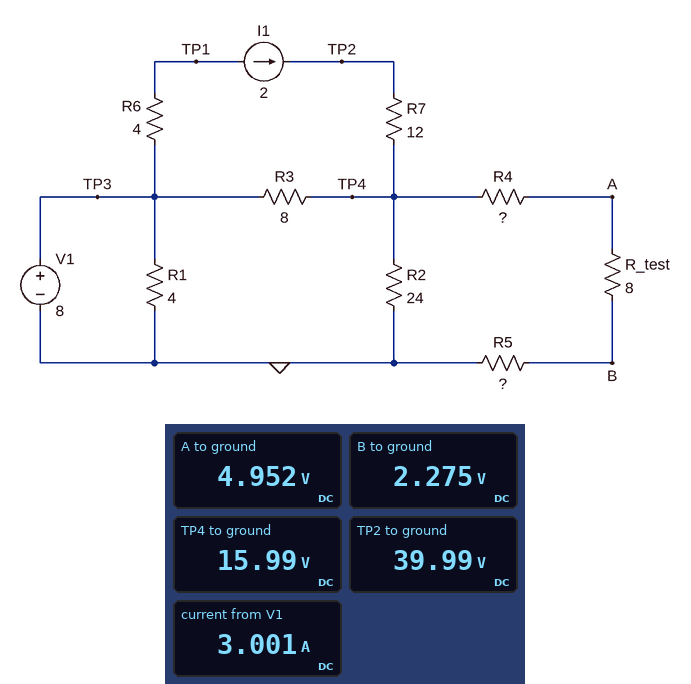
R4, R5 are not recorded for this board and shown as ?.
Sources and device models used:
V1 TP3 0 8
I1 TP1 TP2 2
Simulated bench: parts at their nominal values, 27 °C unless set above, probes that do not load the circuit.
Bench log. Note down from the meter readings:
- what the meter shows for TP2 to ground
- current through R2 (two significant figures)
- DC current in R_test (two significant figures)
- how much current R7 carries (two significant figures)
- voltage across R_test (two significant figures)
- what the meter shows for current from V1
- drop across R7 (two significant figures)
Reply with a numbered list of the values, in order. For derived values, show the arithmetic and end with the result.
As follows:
1. 39.99 V
2. (15.99 V) / 24 Ω = 670 mA
3. (4.952 V - 2.275 V) / 8 Ω = 330 mA
4. (39.99 V - 15.99 V) / 12 Ω = 2.0 A
5. 4.952 V - 2.275 V = 2.7 V
6. 3.001 A
7. 39.99 V - 15.99 V = 24 V
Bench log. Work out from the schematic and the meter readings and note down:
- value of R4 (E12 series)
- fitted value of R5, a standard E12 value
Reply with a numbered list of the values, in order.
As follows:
1. 33 Ω
2. 6.8 Ω
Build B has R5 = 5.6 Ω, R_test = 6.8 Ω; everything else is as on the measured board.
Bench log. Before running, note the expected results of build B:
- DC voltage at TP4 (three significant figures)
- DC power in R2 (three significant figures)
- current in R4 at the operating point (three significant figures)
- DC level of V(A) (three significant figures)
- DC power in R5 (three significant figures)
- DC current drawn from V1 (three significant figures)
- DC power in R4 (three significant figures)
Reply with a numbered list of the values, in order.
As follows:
1. 15.9 V
2. 10.5 W
3. 350 mA
4. 4.34 V
5. 687 mW
6. 3.01 A
7. 4.05 W
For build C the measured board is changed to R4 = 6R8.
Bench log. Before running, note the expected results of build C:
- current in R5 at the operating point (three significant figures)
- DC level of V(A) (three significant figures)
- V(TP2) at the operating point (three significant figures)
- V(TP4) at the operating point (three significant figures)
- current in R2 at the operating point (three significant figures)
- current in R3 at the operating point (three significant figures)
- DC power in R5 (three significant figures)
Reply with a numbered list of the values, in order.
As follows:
1. 652 mA
2. 9.65 V
3. 38.1 V
4. 14.1 V
5. 587 mA
6. 761 mA
7. 2.89 W
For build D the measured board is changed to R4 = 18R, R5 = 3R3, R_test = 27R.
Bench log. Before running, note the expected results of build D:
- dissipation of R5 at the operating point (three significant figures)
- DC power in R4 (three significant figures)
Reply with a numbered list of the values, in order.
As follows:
1. 363 mW
2. 1.98 W
